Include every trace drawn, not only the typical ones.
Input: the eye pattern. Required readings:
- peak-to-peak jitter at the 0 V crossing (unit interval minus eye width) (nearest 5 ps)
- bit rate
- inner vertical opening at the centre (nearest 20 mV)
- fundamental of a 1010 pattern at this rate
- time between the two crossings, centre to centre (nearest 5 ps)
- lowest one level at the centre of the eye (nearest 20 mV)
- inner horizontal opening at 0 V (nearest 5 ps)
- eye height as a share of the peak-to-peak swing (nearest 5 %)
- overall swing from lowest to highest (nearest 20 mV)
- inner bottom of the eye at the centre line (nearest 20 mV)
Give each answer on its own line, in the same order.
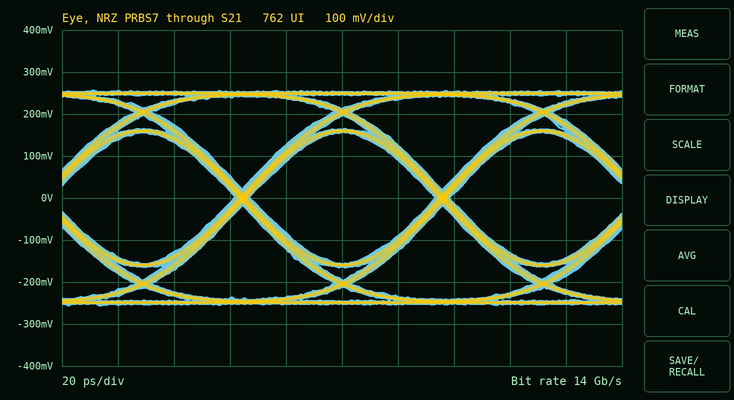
5 ps
14 Gb/s
320 mV
7 GHz
70 ps
160 mV
65 ps
60 %
520 mV
-160 mV
